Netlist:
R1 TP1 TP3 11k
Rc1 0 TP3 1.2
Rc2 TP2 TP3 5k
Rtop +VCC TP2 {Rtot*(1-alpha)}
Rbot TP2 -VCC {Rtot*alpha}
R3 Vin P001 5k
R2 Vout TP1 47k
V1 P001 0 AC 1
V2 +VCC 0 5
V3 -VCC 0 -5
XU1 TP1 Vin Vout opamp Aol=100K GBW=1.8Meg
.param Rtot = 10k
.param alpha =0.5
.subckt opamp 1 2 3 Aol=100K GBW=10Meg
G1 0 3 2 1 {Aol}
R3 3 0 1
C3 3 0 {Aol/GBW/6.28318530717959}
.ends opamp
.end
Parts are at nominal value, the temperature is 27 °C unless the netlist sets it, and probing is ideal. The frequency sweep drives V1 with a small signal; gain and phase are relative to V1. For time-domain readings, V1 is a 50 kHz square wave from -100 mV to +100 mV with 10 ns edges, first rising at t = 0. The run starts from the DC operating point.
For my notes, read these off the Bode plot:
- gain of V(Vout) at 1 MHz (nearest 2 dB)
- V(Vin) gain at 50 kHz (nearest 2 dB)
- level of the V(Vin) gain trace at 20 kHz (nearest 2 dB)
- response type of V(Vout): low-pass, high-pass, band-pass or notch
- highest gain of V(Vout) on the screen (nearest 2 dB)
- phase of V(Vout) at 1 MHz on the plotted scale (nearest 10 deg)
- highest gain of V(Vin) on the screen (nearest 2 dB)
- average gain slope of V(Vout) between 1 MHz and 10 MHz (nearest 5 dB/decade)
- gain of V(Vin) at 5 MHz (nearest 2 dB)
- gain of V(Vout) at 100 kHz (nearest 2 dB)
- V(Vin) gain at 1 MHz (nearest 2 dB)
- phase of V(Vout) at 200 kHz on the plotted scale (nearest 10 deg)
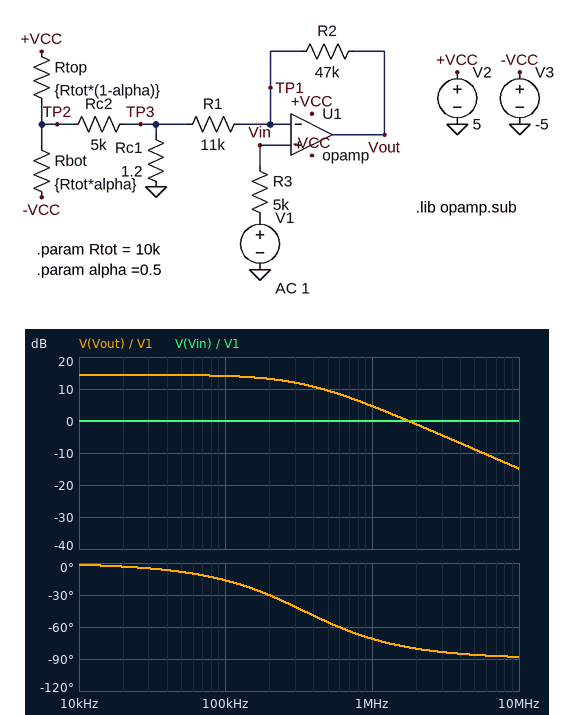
4 dB
0 dB
0 dB
low-pass
14 dB
-70 deg
0 dB
-20 dB/decade
0 dB
14 dB
0 dB
-30 deg
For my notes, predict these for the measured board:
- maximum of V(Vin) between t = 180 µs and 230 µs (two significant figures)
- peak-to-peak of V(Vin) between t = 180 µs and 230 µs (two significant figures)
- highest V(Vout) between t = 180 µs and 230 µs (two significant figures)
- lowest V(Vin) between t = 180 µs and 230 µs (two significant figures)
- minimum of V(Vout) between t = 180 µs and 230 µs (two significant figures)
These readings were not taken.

100 mV
200 mV
530 mV
-100 mV
-530 mV
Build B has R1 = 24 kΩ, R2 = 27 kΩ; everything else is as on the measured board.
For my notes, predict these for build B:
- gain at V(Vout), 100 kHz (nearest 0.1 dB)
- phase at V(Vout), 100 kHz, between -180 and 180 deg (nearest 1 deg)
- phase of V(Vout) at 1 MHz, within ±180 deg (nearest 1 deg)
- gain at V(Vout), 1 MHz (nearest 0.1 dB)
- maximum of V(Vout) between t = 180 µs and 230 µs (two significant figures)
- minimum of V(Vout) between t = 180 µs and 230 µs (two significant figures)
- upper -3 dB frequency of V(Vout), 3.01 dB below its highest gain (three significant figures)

6.5 dB
-7 deg
-50 deg
2.8 dB
210 mV
-210 mV
847 kHz
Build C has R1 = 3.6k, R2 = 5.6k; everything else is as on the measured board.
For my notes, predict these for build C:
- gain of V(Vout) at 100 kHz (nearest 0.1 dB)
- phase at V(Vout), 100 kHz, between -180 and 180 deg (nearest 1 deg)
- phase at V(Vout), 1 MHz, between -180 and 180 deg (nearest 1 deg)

8.1 dB
-8 deg
-55 deg
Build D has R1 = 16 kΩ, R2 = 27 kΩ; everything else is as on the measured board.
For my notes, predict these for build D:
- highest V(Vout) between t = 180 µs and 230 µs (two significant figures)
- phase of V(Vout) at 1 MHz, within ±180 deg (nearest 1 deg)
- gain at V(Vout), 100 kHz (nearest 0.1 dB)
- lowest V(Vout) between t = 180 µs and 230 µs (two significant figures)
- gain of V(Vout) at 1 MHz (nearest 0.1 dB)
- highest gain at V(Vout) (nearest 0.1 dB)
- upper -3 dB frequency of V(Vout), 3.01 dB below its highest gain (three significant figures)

270 mV
-56 deg
8.5 dB
-270 mV
3.5 dB
8.6 dB
670 kHz
